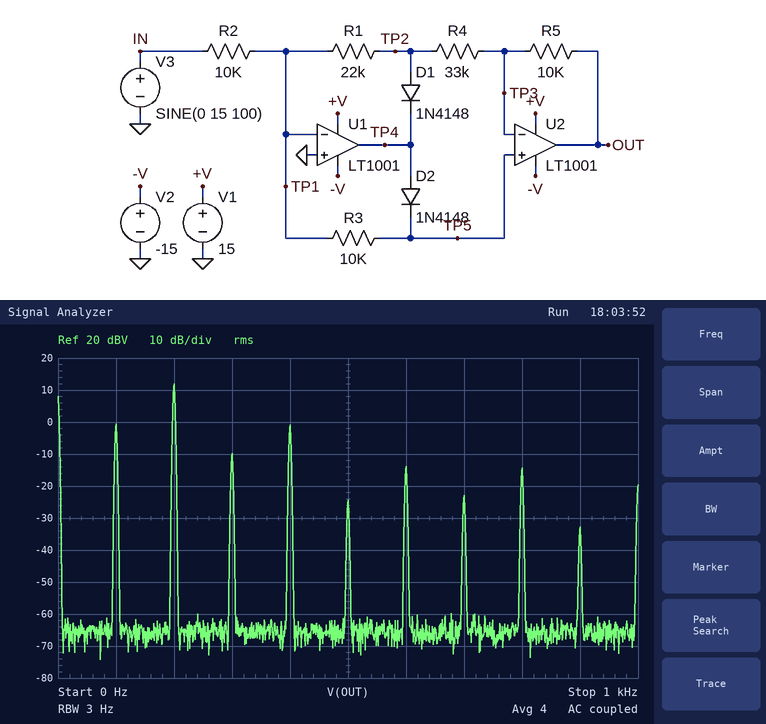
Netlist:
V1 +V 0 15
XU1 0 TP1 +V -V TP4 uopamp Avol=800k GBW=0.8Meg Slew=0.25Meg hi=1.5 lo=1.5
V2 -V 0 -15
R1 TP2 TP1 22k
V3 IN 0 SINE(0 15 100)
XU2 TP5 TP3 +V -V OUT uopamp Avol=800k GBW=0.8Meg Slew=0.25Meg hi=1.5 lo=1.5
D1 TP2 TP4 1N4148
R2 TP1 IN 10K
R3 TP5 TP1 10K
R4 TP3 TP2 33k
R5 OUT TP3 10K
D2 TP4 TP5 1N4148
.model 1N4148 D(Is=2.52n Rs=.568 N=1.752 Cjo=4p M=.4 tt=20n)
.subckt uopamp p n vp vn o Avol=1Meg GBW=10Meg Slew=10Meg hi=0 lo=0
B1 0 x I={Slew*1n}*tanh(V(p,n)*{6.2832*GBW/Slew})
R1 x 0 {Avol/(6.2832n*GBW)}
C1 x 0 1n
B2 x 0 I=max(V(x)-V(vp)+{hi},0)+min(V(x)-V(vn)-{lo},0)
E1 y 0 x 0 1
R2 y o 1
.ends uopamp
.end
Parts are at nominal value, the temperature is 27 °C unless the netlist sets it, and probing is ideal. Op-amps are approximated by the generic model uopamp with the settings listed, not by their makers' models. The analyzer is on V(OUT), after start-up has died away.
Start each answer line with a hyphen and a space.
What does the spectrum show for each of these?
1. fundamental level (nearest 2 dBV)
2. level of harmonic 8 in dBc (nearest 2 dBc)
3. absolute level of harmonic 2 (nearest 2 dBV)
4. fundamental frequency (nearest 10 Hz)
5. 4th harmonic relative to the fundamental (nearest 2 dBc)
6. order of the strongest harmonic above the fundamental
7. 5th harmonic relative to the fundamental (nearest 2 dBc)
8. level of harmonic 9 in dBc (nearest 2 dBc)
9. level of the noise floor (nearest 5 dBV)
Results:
- 0 dBV
- -14 dBc
- 12 dBV
- 100 Hz
- 0 dBc
- 2
- -24 dBc
- -32 dBc
- -65 dBV
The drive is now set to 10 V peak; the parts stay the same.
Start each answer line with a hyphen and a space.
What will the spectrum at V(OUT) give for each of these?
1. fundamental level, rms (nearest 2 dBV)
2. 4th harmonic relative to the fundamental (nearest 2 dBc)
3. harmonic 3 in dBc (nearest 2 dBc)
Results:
- 0 dBV
- -6 dBc
- -18 dBc
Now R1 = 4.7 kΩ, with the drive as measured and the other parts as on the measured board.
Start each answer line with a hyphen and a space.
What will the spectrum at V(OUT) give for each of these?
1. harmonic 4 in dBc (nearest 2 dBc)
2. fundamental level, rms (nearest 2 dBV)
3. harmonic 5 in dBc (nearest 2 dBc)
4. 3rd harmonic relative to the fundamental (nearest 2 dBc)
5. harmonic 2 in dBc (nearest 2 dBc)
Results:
- -16 dBc
- 12 dBV
- -32 dBc
- -28 dBc
- -6 dBc
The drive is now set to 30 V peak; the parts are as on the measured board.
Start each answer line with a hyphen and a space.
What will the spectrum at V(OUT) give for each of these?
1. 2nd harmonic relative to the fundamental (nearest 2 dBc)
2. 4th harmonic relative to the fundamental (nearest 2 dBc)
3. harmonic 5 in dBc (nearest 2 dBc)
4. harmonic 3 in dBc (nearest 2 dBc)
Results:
- 26 dBc
- 24 dBc
- 8 dBc
- 8 dBc
